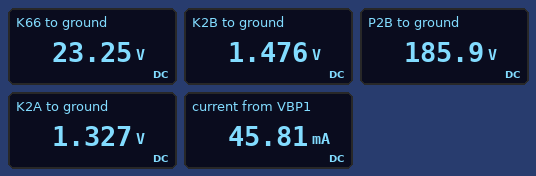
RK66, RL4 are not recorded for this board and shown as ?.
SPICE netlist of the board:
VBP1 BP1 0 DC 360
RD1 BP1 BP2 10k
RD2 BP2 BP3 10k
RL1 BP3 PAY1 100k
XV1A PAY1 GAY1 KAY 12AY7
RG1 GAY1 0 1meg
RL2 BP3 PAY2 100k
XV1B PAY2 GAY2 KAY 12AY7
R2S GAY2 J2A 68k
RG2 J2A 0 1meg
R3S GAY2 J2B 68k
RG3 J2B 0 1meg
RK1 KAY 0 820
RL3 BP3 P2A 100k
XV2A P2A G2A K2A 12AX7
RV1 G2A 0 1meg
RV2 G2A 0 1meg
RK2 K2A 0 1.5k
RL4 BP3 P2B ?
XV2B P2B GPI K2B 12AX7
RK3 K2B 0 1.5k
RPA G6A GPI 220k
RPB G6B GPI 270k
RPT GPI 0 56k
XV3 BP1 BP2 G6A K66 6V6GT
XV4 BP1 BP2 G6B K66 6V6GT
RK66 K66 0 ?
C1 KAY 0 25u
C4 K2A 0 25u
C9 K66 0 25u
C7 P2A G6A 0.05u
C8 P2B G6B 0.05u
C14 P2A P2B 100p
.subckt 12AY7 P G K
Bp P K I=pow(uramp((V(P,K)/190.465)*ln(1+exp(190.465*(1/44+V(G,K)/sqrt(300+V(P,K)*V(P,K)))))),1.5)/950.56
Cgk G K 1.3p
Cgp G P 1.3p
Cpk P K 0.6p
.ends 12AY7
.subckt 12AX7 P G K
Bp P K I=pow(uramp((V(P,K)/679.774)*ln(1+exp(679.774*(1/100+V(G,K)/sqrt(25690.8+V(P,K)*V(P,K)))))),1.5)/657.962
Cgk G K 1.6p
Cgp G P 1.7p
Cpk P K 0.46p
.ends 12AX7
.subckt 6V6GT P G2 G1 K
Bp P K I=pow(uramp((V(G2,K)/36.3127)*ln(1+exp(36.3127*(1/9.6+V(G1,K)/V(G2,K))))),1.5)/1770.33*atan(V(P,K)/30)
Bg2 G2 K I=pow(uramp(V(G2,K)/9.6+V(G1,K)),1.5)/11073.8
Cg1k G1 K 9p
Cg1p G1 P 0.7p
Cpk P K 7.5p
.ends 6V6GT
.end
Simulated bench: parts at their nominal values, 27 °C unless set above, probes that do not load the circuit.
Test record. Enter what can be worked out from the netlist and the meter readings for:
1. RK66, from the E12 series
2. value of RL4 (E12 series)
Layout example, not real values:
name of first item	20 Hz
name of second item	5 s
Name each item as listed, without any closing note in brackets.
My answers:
RK66, from the E12 series	560 Ω
value of RL4	68 kΩ
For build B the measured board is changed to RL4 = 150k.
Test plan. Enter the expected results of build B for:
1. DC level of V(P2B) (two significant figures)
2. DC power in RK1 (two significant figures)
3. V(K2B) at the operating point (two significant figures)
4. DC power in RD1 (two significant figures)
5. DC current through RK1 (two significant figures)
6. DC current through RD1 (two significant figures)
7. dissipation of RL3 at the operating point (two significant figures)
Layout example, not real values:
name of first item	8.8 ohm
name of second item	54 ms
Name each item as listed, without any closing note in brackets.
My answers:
DC level of V(P2B)	140 V
DC power in RK1	5.0 mW
V(K2B) at the operating point	1.2 V
DC power in RD1	390 mW
DC current through RK1	2.5 mA
DC current through RD1	6.3 mA
dissipation of RL3 at the operating point	80 mW
